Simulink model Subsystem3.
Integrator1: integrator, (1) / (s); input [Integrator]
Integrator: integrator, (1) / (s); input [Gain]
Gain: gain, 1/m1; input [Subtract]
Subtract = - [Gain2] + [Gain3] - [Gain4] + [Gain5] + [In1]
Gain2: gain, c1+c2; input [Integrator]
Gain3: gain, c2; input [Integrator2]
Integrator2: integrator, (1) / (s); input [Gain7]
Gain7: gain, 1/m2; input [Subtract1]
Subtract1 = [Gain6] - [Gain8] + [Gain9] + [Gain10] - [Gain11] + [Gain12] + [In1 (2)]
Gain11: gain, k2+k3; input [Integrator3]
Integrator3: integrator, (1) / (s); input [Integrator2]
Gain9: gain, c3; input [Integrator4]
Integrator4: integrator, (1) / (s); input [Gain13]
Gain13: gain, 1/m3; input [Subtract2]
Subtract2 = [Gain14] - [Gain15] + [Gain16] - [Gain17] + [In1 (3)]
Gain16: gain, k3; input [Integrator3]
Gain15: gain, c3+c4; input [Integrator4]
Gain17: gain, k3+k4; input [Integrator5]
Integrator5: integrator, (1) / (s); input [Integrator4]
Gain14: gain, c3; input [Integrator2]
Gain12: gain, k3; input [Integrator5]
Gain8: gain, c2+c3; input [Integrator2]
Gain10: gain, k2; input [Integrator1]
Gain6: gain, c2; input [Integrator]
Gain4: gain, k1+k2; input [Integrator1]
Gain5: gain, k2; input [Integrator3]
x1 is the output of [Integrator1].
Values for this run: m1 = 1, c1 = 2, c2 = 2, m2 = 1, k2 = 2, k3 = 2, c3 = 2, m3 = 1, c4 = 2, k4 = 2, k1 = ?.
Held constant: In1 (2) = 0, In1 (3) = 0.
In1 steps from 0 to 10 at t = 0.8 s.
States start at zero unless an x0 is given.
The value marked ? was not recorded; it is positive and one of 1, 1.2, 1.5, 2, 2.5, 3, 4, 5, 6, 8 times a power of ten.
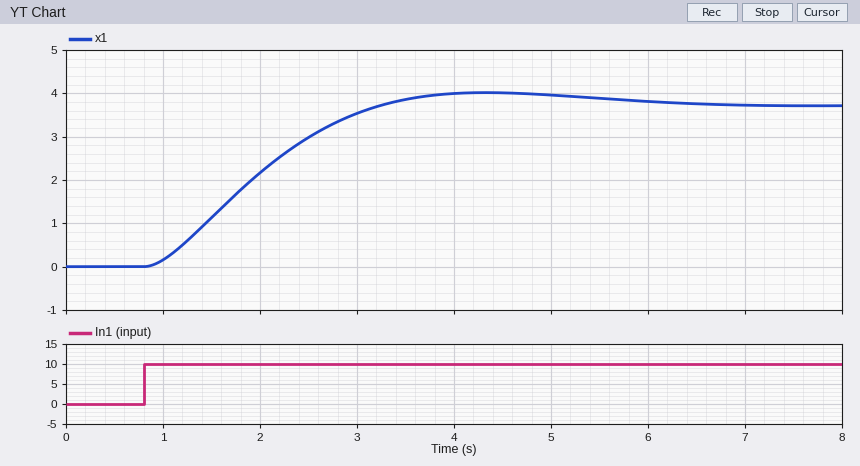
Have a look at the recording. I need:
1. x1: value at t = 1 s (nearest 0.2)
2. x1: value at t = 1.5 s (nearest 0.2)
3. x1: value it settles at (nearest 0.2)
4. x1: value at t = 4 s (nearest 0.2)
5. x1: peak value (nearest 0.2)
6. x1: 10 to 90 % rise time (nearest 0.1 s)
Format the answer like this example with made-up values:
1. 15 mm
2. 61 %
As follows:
1. 0.2
2. 1.2
3. 3.8
4. 4.0
5. 4.0
6. 1.7 s
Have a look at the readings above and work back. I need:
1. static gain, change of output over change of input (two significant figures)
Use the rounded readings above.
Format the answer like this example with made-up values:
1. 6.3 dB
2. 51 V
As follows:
1. 0.38
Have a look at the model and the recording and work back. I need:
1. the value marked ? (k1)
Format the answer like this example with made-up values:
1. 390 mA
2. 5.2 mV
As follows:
1. 2
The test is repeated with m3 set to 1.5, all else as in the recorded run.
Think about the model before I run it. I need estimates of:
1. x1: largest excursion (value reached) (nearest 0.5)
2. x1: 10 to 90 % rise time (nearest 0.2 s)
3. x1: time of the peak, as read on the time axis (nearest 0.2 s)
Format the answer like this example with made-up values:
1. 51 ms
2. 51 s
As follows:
1. 4.0
2. 1.8 s
3. 4.4 s
